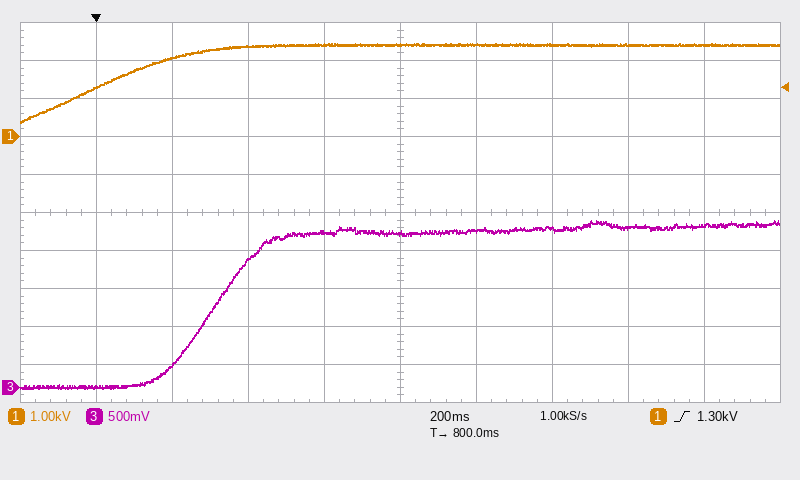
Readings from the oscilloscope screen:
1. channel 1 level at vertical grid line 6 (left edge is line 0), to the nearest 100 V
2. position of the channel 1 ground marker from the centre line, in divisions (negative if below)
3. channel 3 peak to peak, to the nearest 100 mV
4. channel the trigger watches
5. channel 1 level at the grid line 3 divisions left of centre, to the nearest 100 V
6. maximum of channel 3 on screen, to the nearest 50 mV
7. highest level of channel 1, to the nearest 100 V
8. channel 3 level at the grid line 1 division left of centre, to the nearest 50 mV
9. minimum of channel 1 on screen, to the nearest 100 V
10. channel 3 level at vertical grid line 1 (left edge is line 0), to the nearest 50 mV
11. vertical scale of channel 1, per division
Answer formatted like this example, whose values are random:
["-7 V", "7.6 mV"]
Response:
["2.4 kV", "+2.0 div", "2.20 V", "channel 1", "2.1 kV", "2.20 V", "2.4 kV", "2.05 V", "400 V", "0 mV", "1 kV"]
